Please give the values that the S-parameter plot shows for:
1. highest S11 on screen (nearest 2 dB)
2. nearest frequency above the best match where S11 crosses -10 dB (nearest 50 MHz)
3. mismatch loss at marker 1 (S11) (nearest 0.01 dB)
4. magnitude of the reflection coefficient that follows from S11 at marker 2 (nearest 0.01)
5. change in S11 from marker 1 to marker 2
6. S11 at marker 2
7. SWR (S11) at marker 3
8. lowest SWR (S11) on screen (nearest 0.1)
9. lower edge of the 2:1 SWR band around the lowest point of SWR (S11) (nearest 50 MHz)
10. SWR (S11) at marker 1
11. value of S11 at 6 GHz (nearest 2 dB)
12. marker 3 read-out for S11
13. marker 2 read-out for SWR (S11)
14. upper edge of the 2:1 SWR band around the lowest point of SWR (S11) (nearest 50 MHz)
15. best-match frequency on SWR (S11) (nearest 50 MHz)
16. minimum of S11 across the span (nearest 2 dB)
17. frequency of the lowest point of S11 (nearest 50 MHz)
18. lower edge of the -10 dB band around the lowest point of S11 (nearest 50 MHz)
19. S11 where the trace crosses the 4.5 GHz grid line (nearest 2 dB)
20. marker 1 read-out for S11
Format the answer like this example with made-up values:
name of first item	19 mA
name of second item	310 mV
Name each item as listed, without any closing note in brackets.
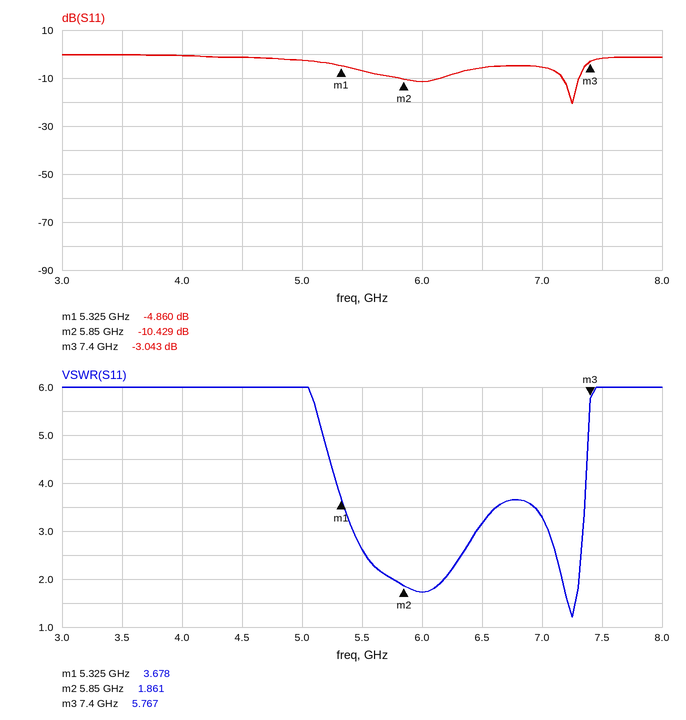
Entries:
highest S11 on screen	0 dB
nearest frequency above the best match where S11 crosses -10 dB	7.30 GHz
mismatch loss at marker 1 (S11)	1.72 dB
magnitude of the reflection coefficient that follows from S11 at marker 2	0.30
change in S11 from marker 1 to marker 2	-5.569 dB
S11 at marker 2	-10.429 dB
SWR (S11) at marker 3	5.767
lowest SWR (S11) on screen	1.2
lower edge of the 2:1 SWR band around the lowest point of SWR (S11)	7.15 GHz
SWR (S11) at marker 1	3.678
value of S11 at 6 GHz	-12 dB
marker 3 read-out for S11	-3.043 dB
marker 2 read-out for SWR	1.861
upper edge of the 2:1 SWR band around the lowest point of SWR (S11)	7.30 GHz
best-match frequency on SWR (S11)	7.25 GHz
minimum of S11 across the span	-20 dB
frequency of the lowest point of S11	7.25 GHz
lower edge of the -10 dB band around the lowest point of S11	7.15 GHz
S11 where the trace crosses the 4.5 GHz grid line	-2 dB
marker 1 read-out for S11	-4.860 dB
